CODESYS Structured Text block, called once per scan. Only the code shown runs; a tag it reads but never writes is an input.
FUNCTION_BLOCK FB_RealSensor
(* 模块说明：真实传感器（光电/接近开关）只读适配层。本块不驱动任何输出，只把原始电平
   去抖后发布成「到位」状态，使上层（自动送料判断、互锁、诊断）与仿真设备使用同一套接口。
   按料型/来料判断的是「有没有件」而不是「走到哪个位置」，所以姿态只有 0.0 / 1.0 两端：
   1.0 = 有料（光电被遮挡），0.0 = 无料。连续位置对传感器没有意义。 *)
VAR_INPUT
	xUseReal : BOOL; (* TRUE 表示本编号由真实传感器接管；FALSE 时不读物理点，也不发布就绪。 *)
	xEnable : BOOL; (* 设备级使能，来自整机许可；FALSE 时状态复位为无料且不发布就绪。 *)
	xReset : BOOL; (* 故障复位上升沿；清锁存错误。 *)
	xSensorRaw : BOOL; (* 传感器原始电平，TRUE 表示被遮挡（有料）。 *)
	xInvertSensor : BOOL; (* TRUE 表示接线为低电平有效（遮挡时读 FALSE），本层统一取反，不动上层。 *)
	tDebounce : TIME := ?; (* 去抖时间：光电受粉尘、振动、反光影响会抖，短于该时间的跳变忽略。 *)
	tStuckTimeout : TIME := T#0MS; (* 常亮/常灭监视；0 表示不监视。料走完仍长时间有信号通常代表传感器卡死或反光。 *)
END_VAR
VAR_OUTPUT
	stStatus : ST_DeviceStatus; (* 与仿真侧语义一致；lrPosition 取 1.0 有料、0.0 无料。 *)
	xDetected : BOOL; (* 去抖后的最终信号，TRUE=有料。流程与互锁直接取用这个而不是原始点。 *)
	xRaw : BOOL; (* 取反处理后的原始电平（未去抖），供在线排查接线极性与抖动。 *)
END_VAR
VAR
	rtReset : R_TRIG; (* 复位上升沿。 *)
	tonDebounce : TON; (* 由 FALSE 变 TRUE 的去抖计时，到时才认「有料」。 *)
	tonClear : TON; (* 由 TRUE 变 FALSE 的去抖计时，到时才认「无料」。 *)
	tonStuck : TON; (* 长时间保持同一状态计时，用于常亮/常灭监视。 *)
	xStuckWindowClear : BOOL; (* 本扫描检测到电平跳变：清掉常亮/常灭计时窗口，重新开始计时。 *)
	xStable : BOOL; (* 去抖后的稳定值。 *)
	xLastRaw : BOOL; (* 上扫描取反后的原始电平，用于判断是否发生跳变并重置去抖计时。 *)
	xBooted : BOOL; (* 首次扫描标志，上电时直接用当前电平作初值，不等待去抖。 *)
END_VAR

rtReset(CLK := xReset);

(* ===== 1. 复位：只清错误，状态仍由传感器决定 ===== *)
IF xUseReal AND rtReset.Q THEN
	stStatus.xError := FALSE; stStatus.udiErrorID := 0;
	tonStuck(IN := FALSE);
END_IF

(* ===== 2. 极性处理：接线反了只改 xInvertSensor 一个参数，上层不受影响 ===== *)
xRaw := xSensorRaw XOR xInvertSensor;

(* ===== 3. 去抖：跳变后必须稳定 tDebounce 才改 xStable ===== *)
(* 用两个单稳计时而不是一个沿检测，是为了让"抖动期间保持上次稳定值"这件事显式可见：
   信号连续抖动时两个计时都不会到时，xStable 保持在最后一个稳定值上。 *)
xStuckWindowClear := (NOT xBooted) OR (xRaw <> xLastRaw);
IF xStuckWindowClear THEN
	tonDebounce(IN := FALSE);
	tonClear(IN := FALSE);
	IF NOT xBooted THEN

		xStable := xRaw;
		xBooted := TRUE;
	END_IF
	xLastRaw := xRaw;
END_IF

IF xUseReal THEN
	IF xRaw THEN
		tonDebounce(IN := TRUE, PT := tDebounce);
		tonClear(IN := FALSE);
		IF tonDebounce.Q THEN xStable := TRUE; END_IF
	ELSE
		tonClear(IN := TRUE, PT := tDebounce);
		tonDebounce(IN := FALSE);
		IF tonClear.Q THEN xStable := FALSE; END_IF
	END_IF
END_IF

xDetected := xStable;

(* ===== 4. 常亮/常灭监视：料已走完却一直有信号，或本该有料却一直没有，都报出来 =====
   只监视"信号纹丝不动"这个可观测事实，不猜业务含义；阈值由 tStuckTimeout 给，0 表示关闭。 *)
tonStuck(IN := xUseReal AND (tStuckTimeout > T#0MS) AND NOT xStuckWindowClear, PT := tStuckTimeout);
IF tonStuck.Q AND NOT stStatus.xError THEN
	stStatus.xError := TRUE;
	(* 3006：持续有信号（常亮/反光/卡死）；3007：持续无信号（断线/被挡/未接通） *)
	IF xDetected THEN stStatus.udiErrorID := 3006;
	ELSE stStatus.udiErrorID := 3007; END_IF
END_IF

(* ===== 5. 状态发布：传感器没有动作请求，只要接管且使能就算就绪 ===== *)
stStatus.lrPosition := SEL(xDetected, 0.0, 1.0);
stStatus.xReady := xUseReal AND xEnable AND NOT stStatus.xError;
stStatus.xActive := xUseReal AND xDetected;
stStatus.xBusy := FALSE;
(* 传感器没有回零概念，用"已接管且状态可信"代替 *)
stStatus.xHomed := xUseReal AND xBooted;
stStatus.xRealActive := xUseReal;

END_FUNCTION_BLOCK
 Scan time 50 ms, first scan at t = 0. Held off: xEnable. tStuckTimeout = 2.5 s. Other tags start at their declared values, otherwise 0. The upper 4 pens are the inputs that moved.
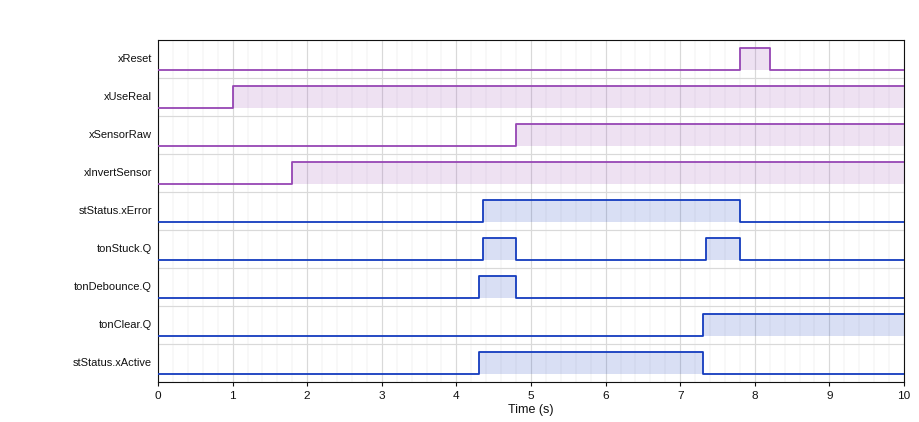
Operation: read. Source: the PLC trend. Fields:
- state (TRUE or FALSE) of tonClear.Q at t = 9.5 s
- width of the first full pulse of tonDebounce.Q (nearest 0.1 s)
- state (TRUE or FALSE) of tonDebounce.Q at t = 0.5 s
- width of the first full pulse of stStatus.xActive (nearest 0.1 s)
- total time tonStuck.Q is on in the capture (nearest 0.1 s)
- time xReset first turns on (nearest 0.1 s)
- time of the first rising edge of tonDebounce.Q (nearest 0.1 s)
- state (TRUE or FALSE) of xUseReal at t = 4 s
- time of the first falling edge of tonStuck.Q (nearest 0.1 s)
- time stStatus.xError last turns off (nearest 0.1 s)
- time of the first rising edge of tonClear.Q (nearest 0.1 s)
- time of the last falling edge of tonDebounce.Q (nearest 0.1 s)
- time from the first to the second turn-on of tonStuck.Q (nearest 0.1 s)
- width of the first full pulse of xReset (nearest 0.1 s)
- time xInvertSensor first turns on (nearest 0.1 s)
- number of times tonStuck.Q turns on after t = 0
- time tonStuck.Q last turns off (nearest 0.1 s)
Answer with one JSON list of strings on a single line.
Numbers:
["TRUE", "0.5 s", "FALSE", "3.0 s", "0.9 s", "7.8 s", "4.3 s", "TRUE", "4.8 s", "7.8 s", "7.3 s", "4.8 s", "3.0 s", "0.4 s", "1.8 s", "2", "7.8 s"]
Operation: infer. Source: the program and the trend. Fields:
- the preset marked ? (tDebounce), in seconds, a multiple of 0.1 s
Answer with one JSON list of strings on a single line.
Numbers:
["2.5 s"]
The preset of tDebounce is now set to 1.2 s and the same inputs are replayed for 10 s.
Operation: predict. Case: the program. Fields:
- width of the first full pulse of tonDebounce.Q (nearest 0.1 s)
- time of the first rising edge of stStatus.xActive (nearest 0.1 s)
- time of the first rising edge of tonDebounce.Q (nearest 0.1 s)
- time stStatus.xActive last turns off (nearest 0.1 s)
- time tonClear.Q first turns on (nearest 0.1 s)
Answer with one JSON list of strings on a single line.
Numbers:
["1.8 s", "3.0 s", "3.0 s", "6.0 s", "6.0 s"]
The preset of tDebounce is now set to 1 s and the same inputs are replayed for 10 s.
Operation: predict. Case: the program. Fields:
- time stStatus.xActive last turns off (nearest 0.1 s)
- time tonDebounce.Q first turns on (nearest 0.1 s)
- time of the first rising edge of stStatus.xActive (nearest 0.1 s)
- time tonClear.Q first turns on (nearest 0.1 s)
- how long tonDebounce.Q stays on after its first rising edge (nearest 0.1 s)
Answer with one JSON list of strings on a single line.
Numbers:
["5.8 s", "2.8 s", "2.8 s", "5.8 s", "2.0 s"]
